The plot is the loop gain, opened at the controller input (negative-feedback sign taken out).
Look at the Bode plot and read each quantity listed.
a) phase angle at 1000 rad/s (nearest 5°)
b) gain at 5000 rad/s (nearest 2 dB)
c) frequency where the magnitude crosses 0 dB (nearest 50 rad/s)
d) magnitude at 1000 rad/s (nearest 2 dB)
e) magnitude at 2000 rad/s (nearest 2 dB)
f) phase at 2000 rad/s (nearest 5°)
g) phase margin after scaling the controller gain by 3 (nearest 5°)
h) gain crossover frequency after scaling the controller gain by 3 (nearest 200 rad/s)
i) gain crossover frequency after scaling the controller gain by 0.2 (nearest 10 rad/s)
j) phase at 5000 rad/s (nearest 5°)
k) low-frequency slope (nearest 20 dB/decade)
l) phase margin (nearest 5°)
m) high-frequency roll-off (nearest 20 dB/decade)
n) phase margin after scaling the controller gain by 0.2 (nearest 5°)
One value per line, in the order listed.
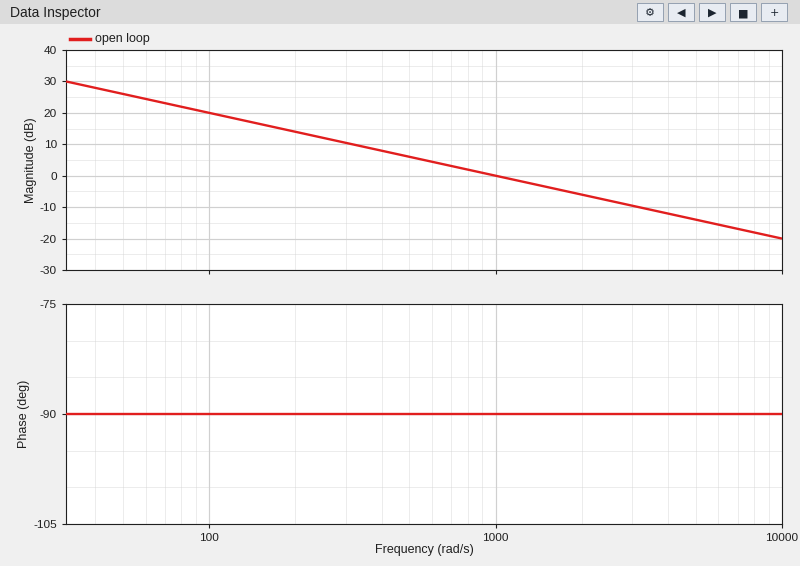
-90°
-14 dB
1000 rad/s
0 dB
-6 dB
-90°
90°
3000 rad/s
200 rad/s
-90°
-20 dB/decade
90°
-20 dB/decade
90°
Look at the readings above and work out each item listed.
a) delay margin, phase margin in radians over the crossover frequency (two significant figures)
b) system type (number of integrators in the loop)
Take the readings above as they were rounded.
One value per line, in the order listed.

0.0016 s
1
